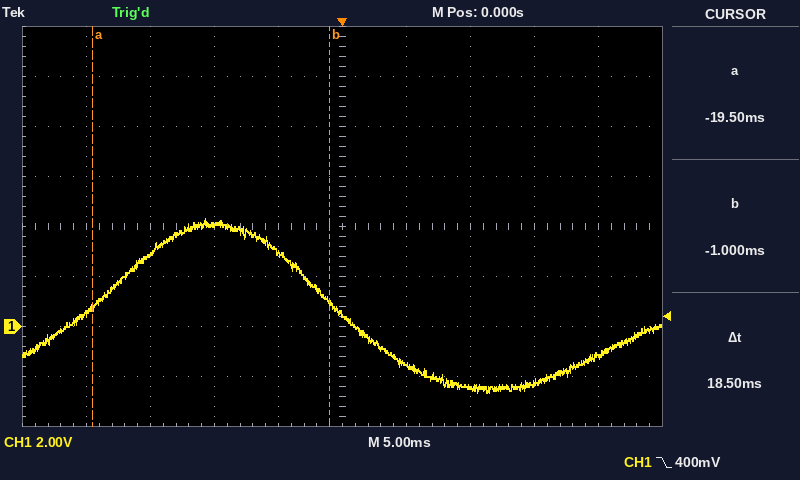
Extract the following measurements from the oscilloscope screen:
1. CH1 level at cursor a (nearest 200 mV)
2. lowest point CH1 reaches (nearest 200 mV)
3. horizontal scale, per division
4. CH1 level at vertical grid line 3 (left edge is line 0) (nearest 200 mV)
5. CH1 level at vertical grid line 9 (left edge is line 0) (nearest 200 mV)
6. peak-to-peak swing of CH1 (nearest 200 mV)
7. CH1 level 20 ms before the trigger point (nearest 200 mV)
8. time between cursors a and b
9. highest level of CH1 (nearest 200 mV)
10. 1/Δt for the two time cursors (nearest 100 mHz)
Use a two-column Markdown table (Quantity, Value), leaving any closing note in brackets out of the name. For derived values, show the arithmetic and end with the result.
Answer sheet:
| Quantity | Value |
|---|---|
| CH1 level at cursor a | 800 mV |
| lowest point CH1 reaches | -2.6 V |
| horizontal scale, per division | 5 ms |
| CH1 level at vertical grid line 3 (left edge is line 0) | 4.0 V |
| CH1 level at vertical grid line 9 (left edge is line 0) | -1.2 V |
| peak-to-peak swing of CH1 | 4.4 V − (-2.6 V) = 7.0 V |
| CH1 level 20 ms before the trigger point | 600 mV |
| time between cursors a and b | 18.5 ms |
| highest level of CH1 | 4.4 V |
| 1/Δt for the two time cursors | 1 / 18.5 ms ≈ 54.1 Hz |
